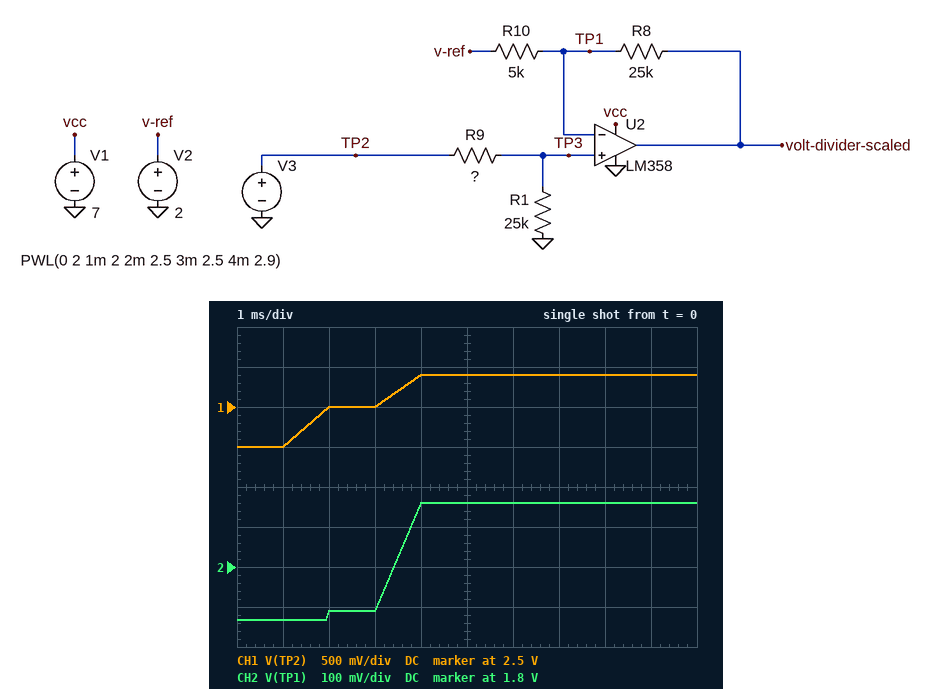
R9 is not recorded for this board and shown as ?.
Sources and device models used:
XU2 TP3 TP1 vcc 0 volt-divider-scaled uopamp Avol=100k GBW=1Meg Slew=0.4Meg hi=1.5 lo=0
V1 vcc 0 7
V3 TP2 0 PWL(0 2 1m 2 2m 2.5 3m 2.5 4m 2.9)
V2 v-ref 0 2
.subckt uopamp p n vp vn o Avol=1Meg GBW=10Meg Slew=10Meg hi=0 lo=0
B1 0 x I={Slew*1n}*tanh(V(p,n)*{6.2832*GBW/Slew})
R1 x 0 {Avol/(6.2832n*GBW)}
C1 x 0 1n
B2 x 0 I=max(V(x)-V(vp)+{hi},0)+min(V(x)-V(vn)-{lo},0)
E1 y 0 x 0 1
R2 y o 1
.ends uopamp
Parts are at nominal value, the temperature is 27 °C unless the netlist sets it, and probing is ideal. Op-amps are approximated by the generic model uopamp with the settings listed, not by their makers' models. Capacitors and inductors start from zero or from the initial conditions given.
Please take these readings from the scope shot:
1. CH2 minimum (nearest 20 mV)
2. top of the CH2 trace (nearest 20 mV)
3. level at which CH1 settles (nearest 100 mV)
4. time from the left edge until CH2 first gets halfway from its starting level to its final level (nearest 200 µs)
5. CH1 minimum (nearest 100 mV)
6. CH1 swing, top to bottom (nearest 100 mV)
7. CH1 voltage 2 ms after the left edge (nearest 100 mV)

1.66 V
1.96 V
2.9 V
3.4 ms
2.0 V
900 mV
2.5 V
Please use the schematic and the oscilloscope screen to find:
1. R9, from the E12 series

12 kΩ
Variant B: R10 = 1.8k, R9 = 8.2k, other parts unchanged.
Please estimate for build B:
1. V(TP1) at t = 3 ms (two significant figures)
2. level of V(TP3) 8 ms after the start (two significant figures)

1.9 V
2.2 V
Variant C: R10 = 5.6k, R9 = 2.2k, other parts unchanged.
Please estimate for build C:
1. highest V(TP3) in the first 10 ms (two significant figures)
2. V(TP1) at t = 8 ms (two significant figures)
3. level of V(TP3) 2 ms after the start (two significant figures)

2.7 V
2.6 V
2.3 V
